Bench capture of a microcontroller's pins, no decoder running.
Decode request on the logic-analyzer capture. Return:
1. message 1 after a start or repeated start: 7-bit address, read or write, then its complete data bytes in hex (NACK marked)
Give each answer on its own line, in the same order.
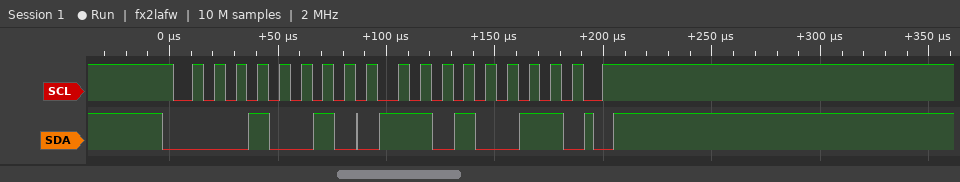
0x09 write: D3
